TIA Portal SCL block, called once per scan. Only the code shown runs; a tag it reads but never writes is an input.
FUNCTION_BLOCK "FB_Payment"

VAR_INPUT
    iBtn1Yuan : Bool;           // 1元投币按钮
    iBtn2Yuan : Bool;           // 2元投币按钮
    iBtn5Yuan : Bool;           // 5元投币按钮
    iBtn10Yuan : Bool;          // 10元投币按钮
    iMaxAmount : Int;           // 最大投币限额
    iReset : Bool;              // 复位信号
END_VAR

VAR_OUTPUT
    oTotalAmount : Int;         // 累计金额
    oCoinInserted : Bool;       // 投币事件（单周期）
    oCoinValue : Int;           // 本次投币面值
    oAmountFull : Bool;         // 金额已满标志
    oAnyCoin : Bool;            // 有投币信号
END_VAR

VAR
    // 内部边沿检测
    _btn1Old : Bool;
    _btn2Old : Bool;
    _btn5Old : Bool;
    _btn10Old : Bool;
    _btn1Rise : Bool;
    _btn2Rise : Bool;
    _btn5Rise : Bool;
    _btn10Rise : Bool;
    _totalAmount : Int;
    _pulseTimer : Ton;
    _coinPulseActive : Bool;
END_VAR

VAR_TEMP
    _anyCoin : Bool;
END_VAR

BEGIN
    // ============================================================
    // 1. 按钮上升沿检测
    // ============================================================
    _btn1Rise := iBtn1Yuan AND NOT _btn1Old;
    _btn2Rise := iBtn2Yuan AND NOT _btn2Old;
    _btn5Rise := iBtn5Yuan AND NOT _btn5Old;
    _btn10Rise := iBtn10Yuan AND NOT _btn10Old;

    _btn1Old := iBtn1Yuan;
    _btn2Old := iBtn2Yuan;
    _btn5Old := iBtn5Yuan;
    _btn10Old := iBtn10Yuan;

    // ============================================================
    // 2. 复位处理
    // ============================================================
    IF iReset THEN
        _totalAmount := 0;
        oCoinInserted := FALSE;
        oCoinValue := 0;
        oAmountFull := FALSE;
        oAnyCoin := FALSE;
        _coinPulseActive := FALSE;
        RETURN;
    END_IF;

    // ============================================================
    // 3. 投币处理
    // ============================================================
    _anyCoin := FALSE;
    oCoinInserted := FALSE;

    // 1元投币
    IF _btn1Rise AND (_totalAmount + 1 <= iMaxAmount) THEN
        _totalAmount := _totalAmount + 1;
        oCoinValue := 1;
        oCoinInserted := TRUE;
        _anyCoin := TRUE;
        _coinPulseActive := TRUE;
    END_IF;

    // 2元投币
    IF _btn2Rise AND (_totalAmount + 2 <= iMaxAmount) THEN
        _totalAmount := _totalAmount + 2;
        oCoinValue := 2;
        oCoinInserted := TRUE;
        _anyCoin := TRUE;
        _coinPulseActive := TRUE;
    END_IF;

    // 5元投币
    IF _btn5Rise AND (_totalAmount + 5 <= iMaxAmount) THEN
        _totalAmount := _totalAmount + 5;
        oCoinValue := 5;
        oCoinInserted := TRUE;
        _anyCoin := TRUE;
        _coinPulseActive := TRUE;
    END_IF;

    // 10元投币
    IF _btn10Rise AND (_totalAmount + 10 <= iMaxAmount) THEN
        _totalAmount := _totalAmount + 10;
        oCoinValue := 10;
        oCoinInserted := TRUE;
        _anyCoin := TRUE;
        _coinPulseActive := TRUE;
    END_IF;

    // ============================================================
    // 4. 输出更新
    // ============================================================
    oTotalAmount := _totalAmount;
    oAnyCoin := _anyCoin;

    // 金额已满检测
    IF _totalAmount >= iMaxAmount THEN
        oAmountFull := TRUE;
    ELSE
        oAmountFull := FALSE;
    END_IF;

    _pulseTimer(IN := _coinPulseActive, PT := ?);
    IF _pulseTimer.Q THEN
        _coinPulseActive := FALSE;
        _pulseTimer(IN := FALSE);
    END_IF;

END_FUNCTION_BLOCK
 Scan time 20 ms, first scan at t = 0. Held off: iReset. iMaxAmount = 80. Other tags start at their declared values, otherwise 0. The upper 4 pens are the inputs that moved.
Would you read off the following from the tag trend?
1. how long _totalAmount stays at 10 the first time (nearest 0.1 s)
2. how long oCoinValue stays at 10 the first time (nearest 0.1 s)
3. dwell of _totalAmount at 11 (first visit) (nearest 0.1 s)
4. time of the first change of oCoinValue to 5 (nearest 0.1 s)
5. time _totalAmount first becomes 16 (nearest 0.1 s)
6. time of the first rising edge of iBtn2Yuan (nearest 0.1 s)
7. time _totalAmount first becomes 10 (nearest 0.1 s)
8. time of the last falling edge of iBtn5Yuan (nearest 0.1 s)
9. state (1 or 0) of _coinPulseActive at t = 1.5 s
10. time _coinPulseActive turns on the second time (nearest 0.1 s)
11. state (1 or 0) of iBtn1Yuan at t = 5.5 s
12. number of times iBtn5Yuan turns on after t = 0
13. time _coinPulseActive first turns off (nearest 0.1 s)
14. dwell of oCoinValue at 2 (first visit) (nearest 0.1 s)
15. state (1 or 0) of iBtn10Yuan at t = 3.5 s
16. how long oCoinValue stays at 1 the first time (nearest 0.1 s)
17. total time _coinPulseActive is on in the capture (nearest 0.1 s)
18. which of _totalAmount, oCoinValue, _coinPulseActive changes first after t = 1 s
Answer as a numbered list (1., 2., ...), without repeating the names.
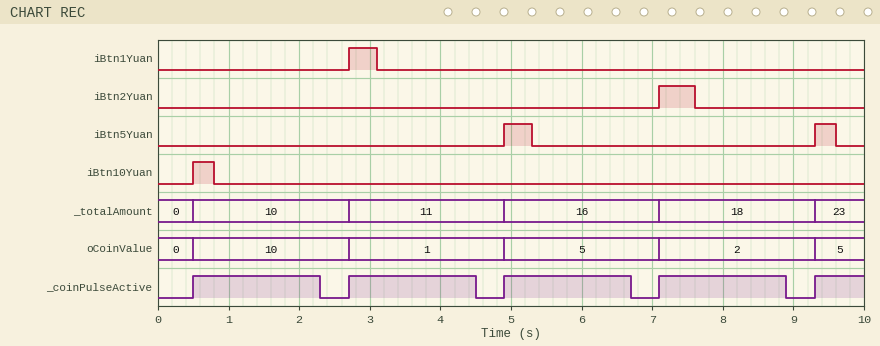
1. 2.2 s
2. 2.2 s
3. 2.2 s
4. 4.9 s
5. 4.9 s
6. 7.1 s
7. 0.5 s
8. 9.6 s
9. 1
10. 2.7 s
11. 0
12. 2
13. 2.3 s
14. 2.2 s
15. 0
16. 2.2 s
17. 7.9 s
18. _coinPulseActive
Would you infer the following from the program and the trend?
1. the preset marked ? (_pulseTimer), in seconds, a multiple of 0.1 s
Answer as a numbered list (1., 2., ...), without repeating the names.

1. 1.8 s
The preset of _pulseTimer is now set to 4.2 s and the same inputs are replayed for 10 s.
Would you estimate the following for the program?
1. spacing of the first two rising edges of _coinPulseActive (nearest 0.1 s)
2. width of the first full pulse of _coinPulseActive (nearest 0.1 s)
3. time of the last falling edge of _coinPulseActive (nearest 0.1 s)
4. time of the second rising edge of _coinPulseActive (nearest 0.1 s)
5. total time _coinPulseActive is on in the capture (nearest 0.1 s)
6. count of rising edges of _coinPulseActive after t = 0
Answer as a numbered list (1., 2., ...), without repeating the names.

1. 4.4 s
2. 4.2 s
3. 9.1 s
4. 4.9 s
5. 9.1 s
6. 3
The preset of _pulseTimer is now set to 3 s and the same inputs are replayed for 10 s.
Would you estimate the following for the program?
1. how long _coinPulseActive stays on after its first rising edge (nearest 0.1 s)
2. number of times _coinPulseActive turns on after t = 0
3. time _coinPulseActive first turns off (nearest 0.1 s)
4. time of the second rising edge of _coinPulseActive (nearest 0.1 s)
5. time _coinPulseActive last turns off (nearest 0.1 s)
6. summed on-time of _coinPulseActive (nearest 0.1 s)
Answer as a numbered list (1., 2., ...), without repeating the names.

1. 3.0 s
2. 3
3. 3.5 s
4. 4.9 s
5. 7.9 s
6. 6.7 s
